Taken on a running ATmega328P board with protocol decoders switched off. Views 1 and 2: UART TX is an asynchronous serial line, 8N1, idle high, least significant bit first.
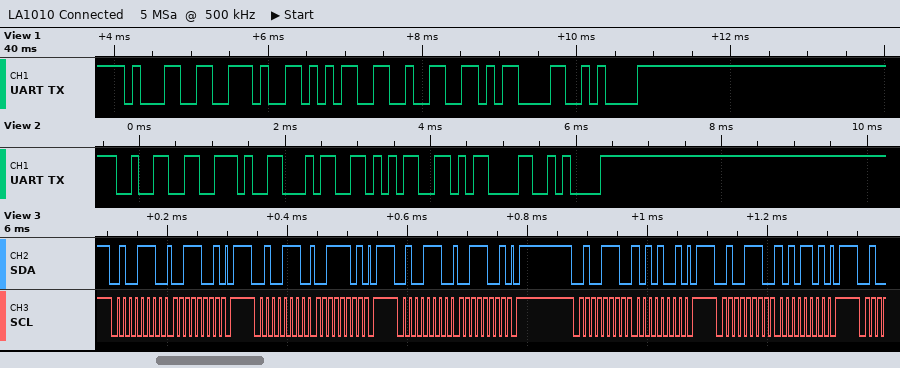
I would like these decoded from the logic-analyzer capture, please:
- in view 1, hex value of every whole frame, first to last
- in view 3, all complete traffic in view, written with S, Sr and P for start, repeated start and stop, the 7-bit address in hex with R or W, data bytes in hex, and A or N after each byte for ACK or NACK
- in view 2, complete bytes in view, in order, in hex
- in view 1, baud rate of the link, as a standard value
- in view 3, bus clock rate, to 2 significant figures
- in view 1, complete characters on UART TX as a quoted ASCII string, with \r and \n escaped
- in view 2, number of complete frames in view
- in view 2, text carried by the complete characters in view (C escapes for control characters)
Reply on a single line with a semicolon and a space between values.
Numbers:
0x31 0x2E 0x35 0x32 0x0D 0x0A; S 27W A 39 A P S 27W A 3D A P S 27W A 39 A P S 27W A A9 A P S 27W A AD A P; 0x32 0x2E 0x34 0x35 0x0D 0x0A; 9600 baud; 100 kHz; "1.52\r\n"; 6; "2.45\r\n"
